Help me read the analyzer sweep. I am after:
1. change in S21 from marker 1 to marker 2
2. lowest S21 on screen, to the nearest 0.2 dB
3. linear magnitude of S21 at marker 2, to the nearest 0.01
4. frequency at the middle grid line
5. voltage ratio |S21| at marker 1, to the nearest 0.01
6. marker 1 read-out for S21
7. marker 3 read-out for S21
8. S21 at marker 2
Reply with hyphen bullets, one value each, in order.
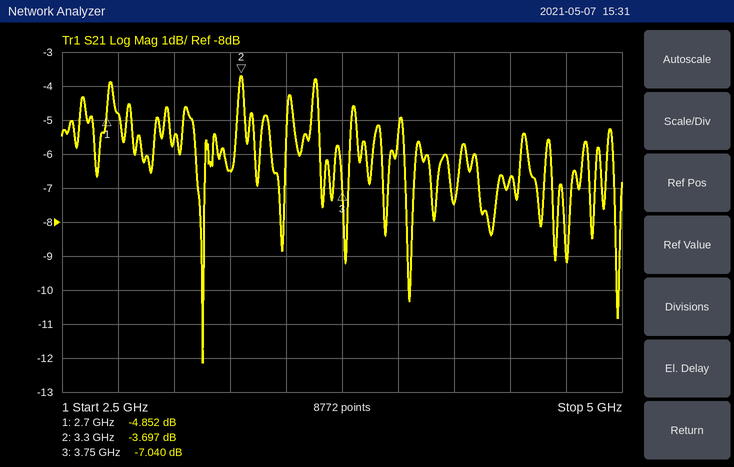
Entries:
- 1.155 dB
- -12.2 dB
- 0.65
- 3.75 GHz
- 0.57
- -4.852 dB
- -7.040 dB
- -3.697 dB
